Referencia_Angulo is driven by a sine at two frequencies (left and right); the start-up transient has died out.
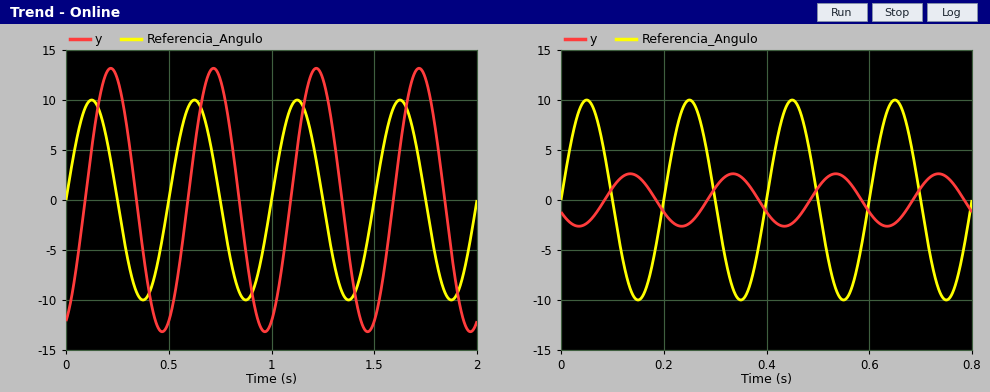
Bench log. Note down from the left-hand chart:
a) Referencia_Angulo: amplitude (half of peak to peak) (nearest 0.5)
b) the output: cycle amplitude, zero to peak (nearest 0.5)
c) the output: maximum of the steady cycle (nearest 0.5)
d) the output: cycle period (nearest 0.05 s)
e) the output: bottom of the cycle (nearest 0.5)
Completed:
10.0
13.0
13.0
0.50 s
-13.0
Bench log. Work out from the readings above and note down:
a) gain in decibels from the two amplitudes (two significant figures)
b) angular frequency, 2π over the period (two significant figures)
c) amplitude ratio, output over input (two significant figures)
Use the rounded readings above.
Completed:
2.3 dB
13 rad/s
1.3
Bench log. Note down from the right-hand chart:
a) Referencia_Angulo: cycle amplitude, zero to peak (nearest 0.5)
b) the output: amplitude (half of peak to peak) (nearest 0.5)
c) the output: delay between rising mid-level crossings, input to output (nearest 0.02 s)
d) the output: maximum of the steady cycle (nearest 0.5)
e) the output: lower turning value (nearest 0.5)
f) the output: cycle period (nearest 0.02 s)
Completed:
10.0
2.5
0.08 s
2.5
-2.5
0.20 s
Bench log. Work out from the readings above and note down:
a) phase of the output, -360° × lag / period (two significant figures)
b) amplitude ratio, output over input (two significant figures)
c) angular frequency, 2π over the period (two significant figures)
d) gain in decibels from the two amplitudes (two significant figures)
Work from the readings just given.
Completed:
-140°
0.25
31 rad/s
-12 dB
